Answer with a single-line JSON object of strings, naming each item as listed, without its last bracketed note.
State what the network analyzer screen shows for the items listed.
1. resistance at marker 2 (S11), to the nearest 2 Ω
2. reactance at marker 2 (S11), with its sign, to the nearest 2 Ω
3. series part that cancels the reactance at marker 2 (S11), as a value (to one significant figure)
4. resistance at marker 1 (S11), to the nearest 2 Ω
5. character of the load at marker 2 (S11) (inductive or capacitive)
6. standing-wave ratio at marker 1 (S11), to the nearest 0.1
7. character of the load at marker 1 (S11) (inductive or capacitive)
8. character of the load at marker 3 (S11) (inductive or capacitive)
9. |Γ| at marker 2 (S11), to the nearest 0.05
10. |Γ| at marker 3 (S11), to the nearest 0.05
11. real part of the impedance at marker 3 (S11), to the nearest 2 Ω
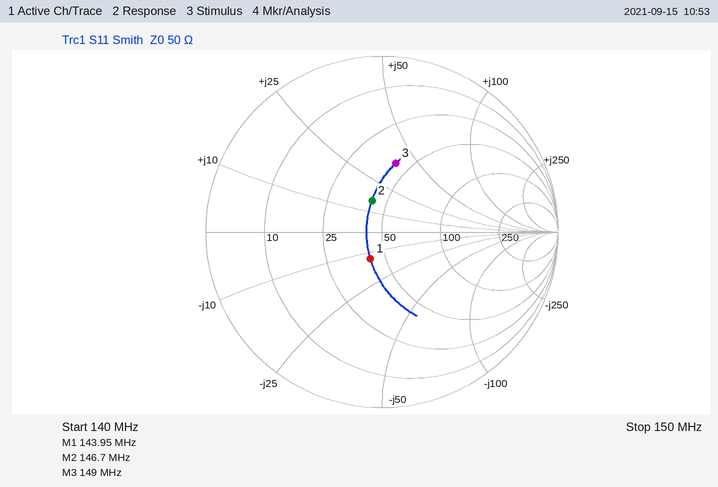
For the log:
{"resistance at marker 2 (S11), to the nearest 2 Ω": "42 Ω", "reactance at marker 2 (S11), with its sign, to the nearest 2 Ω": "+16 Ω", "series part that cancels the reactance at marker 2 (S11), as a value": "70 pF", "resistance at marker 1 (S11), to the nearest 2 Ω": "42 Ω", "character of the load at marker 2 (S11)": "inductive", "standing-wave ratio at marker 1 (S11), to the nearest 0.1": "1.4", "character of the load at marker 1 (S11)": "capacitive", "character of the load at marker 3 (S11)": "inductive", "|Γ| at marker 2 (S11), to the nearest 0.05": "0.20", "|Γ| at marker 3 (S11), to the nearest 0.05": "0.40", "real part of the impedance at marker 3 (S11), to the nearest 2 Ω": "42 Ω"}
